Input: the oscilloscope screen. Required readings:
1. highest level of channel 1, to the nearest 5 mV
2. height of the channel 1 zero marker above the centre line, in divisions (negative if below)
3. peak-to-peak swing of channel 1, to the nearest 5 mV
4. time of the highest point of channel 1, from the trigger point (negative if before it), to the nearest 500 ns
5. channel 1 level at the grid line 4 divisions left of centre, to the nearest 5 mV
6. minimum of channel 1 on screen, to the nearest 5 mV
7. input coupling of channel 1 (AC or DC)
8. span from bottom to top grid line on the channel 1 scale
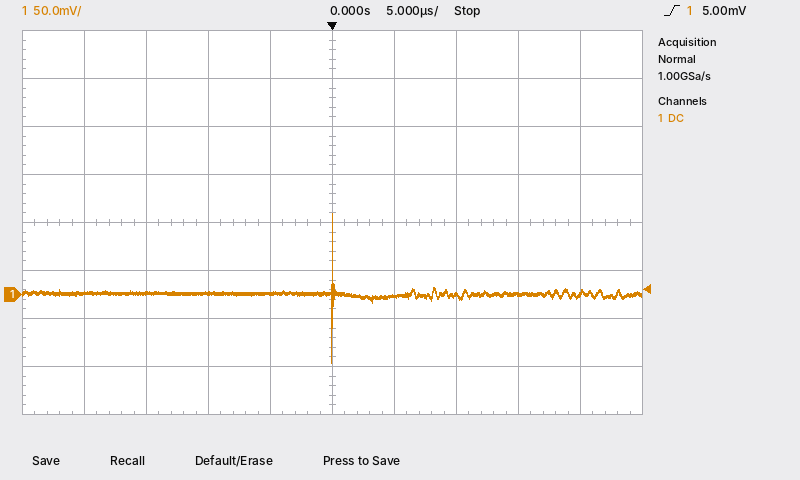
85 mV
-1.5 div
155 mV
0.0 µs
0 mV
-70 mV
DC
400 mV
